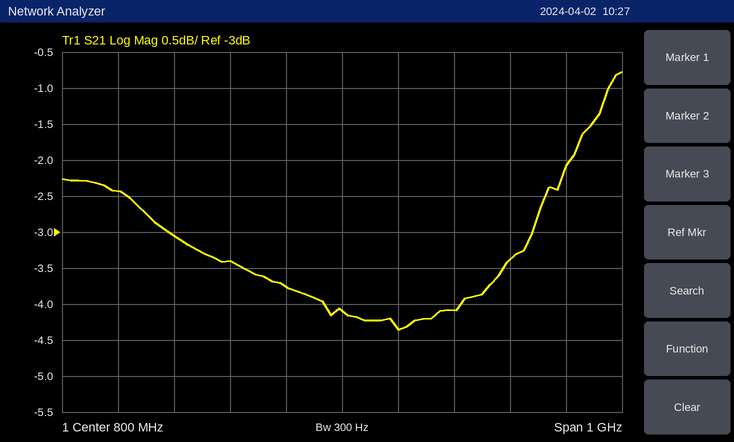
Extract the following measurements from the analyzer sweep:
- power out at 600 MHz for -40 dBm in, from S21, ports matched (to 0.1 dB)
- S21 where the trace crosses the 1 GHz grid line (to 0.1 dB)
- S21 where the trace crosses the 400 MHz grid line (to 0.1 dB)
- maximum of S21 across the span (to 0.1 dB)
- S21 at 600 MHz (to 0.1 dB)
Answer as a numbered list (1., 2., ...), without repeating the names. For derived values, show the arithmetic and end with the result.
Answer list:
1. -40 dBm + (-3.4 dB) = -43.4 dBm
2. -4.1 dB
3. -2.4 dB
4. -0.8 dB
5. -3.4 dB
